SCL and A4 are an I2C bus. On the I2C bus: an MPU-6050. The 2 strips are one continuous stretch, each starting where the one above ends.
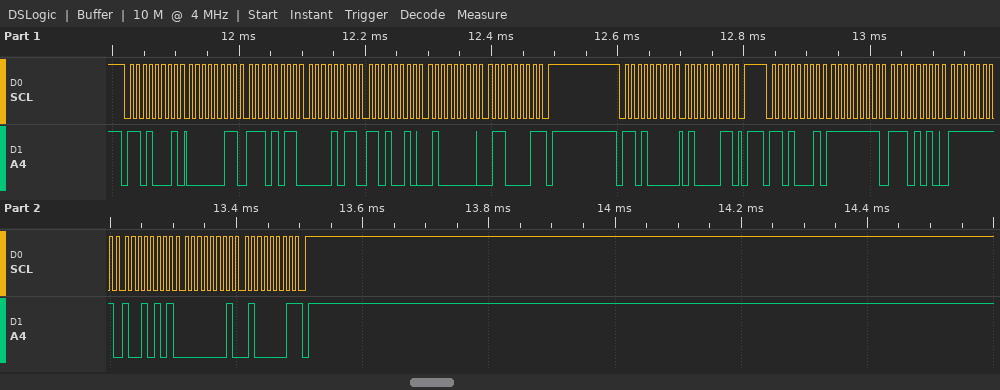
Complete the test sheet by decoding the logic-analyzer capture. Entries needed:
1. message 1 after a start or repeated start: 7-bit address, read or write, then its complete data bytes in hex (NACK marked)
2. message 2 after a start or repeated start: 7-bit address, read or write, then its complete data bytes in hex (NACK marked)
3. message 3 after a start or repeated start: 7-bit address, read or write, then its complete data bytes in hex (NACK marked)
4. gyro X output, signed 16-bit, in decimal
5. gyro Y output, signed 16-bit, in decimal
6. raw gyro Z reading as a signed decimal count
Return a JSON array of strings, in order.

["0x68 read: 03 EB 0B D2 40 61 NACK", "0x68 write: 43", "0x68 read: FF EA FF 95 01 41 NACK", "-22", "-107", "321"]
